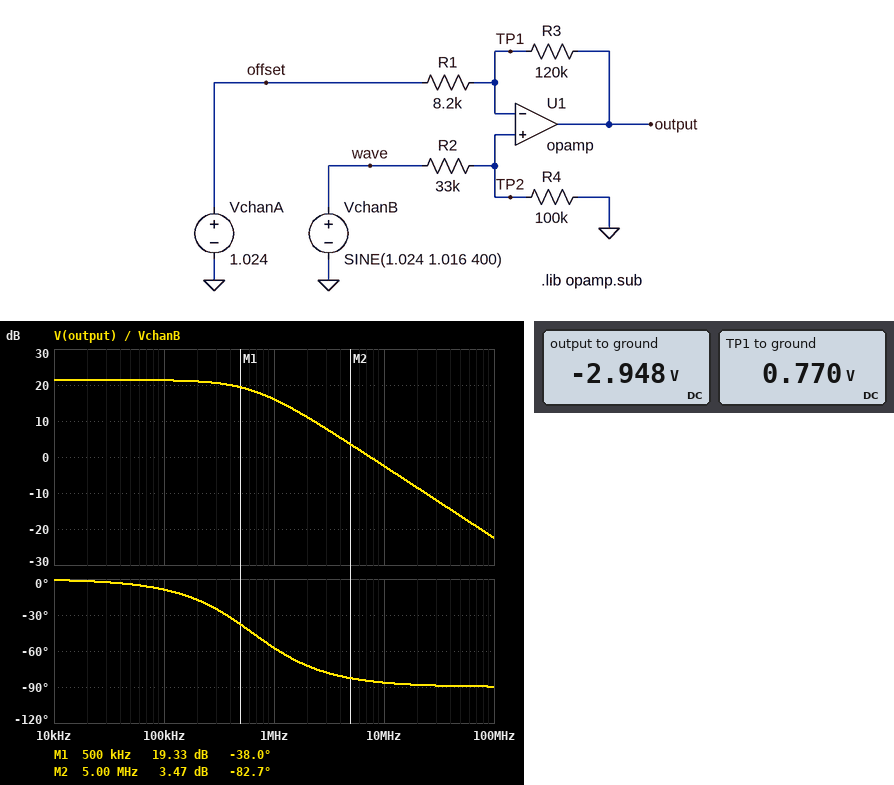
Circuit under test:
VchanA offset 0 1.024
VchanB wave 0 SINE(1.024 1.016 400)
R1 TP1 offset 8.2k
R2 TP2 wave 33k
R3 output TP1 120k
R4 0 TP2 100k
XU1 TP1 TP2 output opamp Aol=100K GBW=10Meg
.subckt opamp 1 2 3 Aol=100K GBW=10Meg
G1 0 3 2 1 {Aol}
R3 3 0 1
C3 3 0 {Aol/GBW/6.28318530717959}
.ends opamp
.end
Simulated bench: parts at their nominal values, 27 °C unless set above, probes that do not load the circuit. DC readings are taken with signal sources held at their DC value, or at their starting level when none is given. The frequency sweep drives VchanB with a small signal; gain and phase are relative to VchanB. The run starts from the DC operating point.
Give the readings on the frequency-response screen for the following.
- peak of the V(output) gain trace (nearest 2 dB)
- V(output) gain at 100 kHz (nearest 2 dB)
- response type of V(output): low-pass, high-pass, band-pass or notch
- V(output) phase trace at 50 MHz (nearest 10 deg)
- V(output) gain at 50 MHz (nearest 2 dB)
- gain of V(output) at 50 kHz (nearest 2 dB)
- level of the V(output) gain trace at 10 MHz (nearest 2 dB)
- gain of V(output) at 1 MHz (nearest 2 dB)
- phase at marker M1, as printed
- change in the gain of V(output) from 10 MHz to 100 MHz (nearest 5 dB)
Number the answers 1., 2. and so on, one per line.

1. 22 dB
2. 22 dB
3. low-pass
4. -90 deg
5. -16 dB
6. 22 dB
7. -2 dB
8. 16 dB
9. -38.0 deg
10. -20 dB
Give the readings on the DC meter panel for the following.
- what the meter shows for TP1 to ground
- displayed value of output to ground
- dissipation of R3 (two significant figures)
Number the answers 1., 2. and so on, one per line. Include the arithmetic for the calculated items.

1. 0.770 V
2. -2.948 V
3. (770 mV - (-2.948 V))^2 / 120 kΩ = 120 µW
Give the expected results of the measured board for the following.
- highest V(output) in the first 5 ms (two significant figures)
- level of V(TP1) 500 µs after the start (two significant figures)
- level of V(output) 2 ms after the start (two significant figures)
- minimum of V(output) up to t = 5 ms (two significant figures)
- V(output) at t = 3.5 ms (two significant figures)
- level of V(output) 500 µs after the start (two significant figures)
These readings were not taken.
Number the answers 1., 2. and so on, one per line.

1. 9.0 V
2. 1.5 V
3. -14 V
4. -15 V
5. 4.1 V
6. 8.4 V
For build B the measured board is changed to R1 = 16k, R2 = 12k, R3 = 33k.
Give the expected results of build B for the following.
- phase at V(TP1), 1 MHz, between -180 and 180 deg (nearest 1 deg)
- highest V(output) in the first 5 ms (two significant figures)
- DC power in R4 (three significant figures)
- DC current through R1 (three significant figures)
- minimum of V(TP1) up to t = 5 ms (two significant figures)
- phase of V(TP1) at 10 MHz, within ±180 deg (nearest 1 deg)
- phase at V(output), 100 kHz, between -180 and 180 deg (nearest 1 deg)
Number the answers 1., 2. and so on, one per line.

1. -17 deg
2. 3.5 V
3. 8.36 µW
4. 6.86 µA
5. 7.2 mV
6. -72 deg
7. -2 deg
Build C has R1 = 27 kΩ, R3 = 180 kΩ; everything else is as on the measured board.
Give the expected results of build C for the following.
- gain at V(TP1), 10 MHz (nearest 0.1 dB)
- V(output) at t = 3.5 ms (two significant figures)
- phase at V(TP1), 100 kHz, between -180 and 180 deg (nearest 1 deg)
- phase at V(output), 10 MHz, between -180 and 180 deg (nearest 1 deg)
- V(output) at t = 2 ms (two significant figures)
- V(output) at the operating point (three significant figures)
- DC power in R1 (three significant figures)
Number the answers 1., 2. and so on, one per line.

1. -20.2 dB
2. 2.5 V
3. -4 deg
4. -83 deg
5. -6.5 V
6. -924 mV
7. 2.39 µW
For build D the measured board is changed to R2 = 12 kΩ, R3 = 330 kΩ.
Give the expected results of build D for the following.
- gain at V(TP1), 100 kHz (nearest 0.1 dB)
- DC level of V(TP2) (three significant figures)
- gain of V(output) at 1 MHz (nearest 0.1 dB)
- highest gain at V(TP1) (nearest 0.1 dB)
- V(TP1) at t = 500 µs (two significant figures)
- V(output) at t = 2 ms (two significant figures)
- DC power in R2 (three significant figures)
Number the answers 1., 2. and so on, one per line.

1. -1.7 dB
2. 914 mV
3. 18.8 dB
4. -1.0 dB
5. 1.8 V
6. -39 V
7. 1.00 µW
